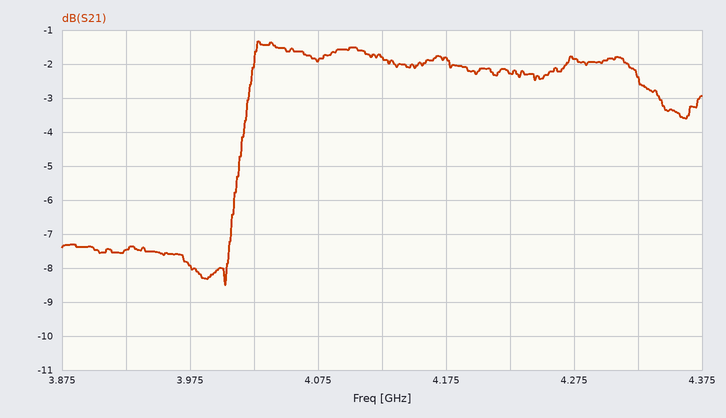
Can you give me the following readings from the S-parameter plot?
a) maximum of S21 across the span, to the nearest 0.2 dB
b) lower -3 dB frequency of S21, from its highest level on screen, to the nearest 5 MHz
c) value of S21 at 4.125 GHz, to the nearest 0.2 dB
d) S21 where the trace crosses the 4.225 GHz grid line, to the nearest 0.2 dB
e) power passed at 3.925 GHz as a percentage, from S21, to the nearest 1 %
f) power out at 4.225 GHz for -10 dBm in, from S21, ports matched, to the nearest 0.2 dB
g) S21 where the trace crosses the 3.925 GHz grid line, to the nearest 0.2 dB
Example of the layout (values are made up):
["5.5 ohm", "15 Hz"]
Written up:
["-1.4 dB", "4.015 GHz", "-1.8 dB", "-2.2 dB", "18 %", "-12.2 dBm", "-7.4 dB"]
